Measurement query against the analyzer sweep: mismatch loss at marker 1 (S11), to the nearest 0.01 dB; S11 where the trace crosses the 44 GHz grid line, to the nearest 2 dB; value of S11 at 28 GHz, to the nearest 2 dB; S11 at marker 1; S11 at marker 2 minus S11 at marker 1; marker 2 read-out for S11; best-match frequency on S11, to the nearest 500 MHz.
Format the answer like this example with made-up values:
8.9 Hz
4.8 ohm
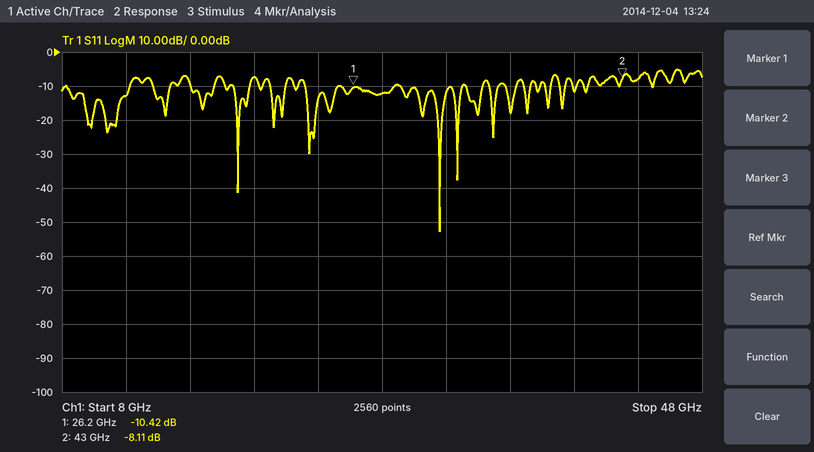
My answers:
0.41 dB
-8 dB
-12 dB
-10.42 dB
2.31 dB
-8.11 dB
31.5 GHz
